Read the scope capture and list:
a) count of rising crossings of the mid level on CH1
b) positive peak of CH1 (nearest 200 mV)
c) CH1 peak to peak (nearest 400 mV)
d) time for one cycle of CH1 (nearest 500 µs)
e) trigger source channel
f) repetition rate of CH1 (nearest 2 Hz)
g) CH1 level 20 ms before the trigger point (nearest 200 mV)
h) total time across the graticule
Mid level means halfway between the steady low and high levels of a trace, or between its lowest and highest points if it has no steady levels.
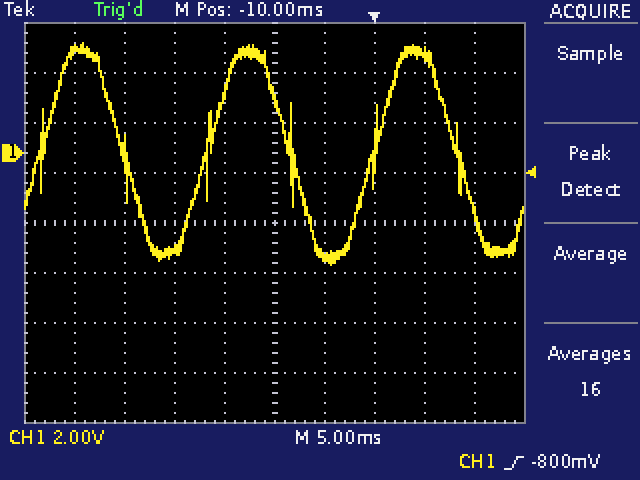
3
4.4 V
8.8 V
16.5 ms
CH1
60 Hz
-3.8 V
50 ms
